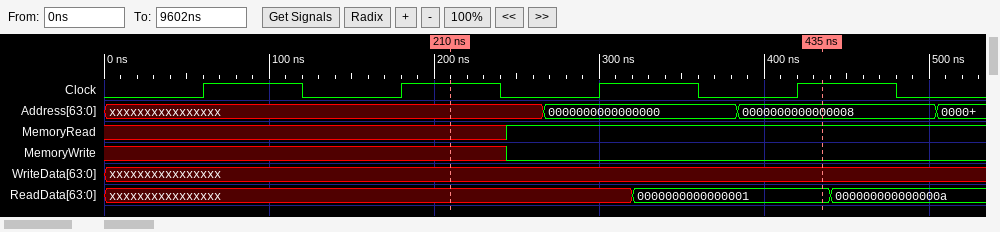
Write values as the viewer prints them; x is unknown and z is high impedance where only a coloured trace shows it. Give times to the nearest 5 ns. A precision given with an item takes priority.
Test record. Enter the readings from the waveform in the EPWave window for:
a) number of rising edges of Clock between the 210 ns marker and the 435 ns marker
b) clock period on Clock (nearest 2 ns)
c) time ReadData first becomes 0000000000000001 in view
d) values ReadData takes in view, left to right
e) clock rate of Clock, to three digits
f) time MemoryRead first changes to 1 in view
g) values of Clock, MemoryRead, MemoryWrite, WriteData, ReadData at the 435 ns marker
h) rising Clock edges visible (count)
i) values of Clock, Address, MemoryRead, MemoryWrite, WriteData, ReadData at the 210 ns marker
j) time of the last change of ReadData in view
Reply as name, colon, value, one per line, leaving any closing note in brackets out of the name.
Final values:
number of rising edges of Clock between the 210 ns marker and the 435 ns marker: 2
clock period on Clock: 120 ns
time ReadData first becomes 0000000000000001 in view: 320 ns
values ReadData takes in view, left to right: xxxxxxxxxxxxxxxx, 0000000000000001, 000000000000000a
clock rate of Clock, to three digits: 8.33 MHz
time MemoryRead first changes to 1 in view: 245 ns
values of Clock, MemoryRead, MemoryWrite, WriteData, ReadData at the 435 ns marker: Clock=1, MemoryRead=1, MemoryWrite=0, WriteData=xxxxxxxxxxxxxxxx, ReadData=0000000000000001
rising Clock edges visible: 4
values of Clock, Address, MemoryRead, MemoryWrite, WriteData, ReadData at the 210 ns marker: Clock=1, Address=xxxxxxxxxxxxxxxx, MemoryRead=x, MemoryWrite=x, WriteData=xxxxxxxxxxxxxxxx, ReadData=xxxxxxxxxxxxxxxx
time of the last change of ReadData in view: 440 ns
